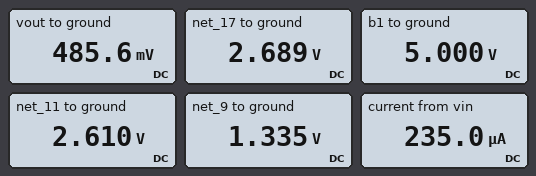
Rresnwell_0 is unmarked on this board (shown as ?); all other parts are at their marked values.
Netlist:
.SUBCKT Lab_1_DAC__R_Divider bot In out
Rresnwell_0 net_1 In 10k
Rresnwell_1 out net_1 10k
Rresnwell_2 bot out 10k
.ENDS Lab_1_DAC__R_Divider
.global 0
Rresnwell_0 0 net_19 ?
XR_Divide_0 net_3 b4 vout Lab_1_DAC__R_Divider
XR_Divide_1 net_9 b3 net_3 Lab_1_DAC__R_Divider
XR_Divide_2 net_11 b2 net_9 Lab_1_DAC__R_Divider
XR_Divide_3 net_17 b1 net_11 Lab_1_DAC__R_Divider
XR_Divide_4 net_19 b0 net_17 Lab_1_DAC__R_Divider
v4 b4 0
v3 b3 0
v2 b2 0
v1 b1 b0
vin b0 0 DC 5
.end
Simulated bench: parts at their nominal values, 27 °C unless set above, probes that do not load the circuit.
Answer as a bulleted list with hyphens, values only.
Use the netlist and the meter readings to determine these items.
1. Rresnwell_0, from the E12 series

- 15 kΩ
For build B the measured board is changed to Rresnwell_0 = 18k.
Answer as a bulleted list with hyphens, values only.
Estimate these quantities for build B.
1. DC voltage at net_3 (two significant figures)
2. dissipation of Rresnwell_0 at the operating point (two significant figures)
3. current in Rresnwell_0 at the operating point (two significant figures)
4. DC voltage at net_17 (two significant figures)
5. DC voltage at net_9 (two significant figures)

- 740 mV
- 180 µW
- 99 µA
- 2.8 V
- 1.4 V
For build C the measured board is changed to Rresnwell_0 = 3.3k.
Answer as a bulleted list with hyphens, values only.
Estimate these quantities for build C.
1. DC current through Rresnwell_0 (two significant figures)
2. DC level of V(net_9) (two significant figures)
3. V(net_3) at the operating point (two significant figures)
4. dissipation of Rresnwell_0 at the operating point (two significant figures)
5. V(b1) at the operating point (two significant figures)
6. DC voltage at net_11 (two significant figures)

- 160 µA
- 1.2 V
- 650 mV
- 86 µW
- 5.0 V
- 2.3 V
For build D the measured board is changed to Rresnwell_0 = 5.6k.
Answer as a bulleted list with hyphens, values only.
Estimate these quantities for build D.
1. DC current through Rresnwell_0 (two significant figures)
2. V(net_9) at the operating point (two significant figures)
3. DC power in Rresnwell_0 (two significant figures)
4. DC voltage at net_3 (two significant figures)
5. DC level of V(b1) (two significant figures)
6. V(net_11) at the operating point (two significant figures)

- 150 µA
- 1.2 V
- 120 µW
- 670 mV
- 5.0 V
- 2.4 V
